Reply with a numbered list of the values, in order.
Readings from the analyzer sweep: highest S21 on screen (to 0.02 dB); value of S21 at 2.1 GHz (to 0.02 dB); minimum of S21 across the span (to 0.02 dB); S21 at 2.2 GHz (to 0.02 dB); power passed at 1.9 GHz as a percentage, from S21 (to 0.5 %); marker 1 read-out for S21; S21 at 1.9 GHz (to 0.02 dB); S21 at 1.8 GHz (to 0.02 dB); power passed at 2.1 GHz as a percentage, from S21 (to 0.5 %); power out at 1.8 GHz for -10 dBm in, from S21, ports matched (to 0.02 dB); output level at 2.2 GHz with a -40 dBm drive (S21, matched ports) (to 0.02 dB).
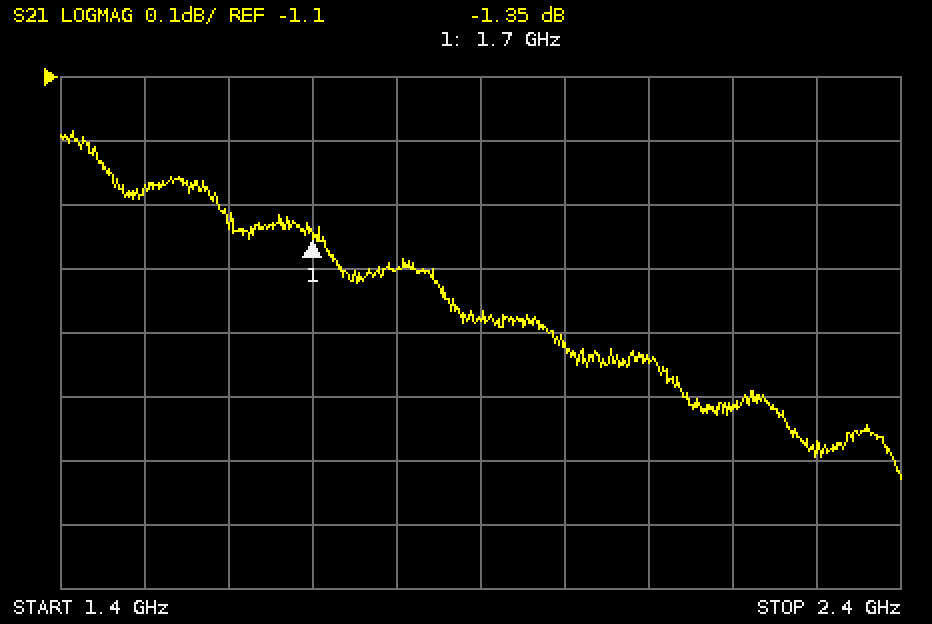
1. -1.18 dB
2. -1.54 dB
3. -1.72 dB
4. -1.62 dB
5. 71.0 %
6. -1.35 dB
7. -1.48 dB
8. -1.40 dB
9. 70.0 %
10. -11.40 dBm
11. -41.62 dBm
